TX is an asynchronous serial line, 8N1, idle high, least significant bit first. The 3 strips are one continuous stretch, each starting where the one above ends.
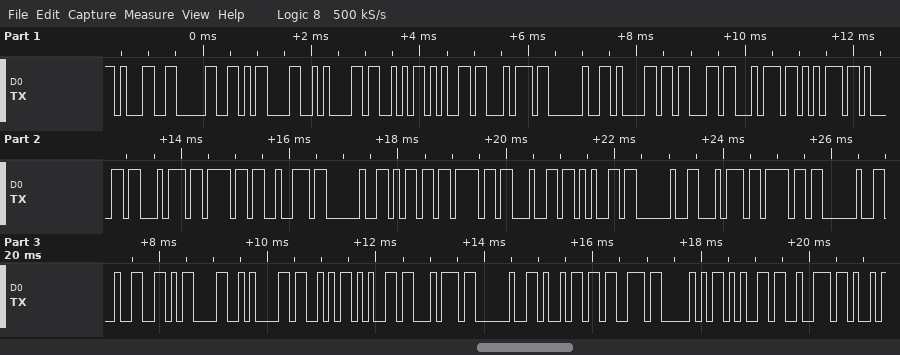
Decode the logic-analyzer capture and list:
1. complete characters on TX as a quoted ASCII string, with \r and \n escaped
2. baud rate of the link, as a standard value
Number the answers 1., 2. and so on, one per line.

1. "10\r\nSet actuator mode to 2\r\nSet isPer"
2. 9600 baud
